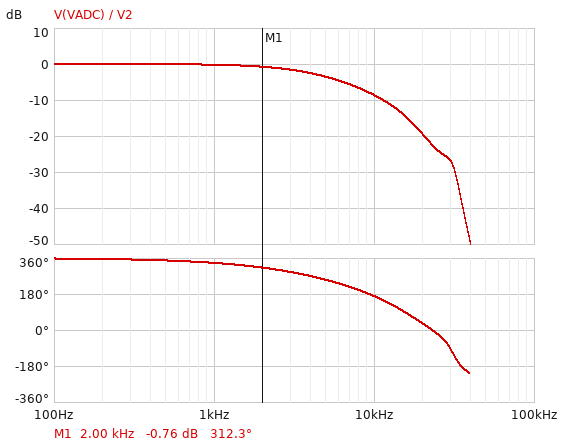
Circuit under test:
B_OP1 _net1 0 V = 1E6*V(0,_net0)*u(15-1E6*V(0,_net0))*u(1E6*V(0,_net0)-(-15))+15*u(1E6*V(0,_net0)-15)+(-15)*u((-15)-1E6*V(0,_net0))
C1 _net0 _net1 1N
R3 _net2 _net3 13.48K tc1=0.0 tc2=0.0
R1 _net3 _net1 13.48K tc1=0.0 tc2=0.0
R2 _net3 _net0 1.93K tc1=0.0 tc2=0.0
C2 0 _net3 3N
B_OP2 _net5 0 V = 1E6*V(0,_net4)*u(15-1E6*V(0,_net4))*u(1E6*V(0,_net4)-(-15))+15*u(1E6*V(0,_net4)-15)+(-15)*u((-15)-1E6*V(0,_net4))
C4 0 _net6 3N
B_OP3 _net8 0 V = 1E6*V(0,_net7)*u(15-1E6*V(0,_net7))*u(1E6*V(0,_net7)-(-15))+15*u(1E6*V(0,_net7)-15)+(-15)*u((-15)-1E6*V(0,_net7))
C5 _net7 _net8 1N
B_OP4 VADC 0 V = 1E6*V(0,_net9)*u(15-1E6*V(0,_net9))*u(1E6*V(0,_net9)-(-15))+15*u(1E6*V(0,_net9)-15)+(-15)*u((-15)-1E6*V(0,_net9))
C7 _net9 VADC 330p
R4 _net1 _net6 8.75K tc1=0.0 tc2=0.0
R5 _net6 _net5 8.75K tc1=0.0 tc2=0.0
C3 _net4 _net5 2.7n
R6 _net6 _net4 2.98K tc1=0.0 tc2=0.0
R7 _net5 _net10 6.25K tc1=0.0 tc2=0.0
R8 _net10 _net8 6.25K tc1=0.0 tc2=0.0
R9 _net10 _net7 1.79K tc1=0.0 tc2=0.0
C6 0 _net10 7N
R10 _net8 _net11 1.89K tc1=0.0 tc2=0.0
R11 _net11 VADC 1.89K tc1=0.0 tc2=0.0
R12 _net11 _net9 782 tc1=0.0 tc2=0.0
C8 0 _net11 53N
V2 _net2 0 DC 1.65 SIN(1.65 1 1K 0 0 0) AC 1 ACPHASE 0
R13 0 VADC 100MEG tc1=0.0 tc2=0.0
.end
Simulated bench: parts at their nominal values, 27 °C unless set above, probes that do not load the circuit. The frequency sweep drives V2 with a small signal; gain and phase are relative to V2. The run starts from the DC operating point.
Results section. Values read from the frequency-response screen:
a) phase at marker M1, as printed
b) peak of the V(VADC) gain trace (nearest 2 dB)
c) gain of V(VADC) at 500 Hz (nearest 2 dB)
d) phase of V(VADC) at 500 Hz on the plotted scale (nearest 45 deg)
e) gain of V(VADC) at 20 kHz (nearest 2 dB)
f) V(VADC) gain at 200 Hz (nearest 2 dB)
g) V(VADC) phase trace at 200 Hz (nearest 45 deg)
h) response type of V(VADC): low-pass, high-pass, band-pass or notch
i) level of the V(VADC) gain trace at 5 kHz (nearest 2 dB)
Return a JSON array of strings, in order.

["312.3 deg", "0 dB", "0 dB", "360 deg", "-20 dB", "0 dB", "360 deg", "low-pass", "-4 dB"]
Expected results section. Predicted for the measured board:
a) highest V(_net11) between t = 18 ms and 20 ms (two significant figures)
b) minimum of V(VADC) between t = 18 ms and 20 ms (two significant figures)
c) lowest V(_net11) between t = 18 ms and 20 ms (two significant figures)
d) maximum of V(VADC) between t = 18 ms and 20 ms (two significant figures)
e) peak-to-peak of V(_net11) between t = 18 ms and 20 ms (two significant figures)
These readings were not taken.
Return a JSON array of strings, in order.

["1.6 mV", "670 mV", "-1.6 mV", "2.6 V", "3.2 mV"]
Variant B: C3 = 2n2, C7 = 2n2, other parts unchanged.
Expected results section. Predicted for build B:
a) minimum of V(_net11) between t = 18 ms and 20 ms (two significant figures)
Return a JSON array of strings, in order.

["-11 mV"]
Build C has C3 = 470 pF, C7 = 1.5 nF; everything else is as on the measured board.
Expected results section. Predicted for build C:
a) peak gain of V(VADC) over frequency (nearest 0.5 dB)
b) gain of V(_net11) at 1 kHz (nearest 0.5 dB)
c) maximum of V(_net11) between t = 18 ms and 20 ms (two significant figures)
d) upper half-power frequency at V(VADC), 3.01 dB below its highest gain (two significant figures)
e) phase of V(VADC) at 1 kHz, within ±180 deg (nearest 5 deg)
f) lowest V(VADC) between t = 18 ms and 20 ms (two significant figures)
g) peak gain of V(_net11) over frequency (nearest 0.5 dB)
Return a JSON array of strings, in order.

["4.0 dB", "-42.5 dB", "7.4 mV", "16 kHz", "-15 deg", "650 mV", "-16.0 dB"]
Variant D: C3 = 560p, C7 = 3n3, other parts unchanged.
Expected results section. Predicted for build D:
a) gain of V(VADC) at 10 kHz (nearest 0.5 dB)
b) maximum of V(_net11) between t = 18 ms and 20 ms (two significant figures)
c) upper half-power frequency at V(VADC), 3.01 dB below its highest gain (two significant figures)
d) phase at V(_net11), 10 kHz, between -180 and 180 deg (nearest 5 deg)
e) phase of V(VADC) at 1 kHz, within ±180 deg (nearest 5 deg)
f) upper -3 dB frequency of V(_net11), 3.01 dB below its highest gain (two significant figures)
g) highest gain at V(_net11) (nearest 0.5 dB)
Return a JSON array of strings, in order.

["1.5 dB", "16 mV", "11 kHz", "45 deg", "-15 deg", "13 kHz", "-14.0 dB"]
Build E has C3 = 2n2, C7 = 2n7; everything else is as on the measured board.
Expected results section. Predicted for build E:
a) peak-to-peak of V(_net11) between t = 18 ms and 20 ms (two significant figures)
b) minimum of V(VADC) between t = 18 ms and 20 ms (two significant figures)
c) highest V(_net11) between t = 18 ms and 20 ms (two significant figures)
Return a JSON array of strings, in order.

["26 mV", "660 mV", "13 mV"]
